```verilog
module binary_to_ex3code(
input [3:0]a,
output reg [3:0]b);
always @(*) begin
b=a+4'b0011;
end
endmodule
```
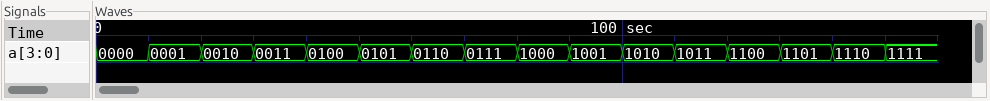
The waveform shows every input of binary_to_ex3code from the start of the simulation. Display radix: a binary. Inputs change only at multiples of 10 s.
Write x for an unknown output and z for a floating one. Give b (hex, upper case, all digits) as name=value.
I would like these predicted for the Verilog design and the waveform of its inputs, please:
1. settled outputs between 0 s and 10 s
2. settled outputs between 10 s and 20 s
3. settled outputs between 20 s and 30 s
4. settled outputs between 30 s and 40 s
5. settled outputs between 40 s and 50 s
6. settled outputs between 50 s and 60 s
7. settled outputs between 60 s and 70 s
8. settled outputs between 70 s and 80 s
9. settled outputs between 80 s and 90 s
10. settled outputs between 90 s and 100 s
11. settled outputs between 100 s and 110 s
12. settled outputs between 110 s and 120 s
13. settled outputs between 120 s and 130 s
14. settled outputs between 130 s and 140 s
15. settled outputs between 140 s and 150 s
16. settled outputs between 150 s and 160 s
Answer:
b=3
b=4
b=5
b=6
b=7
b=8
b=9
b=A
b=B
b=C
b=D
b=E
b=F
b=0
b=1
b=2
